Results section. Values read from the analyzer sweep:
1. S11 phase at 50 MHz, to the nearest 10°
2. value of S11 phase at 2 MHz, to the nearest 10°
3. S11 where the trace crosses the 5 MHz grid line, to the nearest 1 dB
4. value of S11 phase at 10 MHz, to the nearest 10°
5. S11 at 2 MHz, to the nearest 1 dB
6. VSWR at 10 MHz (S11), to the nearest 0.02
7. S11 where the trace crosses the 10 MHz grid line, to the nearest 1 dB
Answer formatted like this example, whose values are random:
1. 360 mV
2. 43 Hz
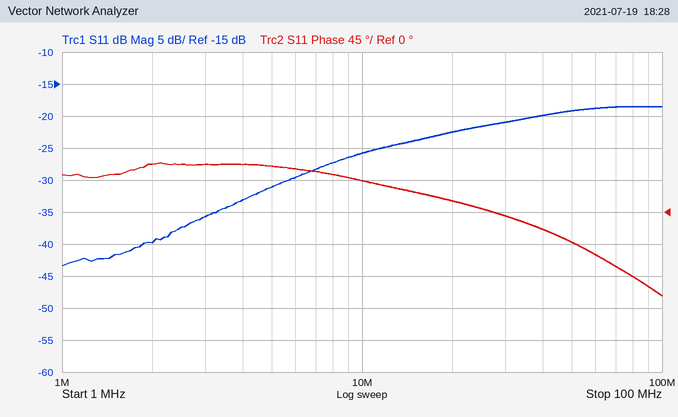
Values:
1. -40°
2. 70°
3. -31 dB
4. 40°
5. -40 dB
6. 1.10
7. -26 dB
